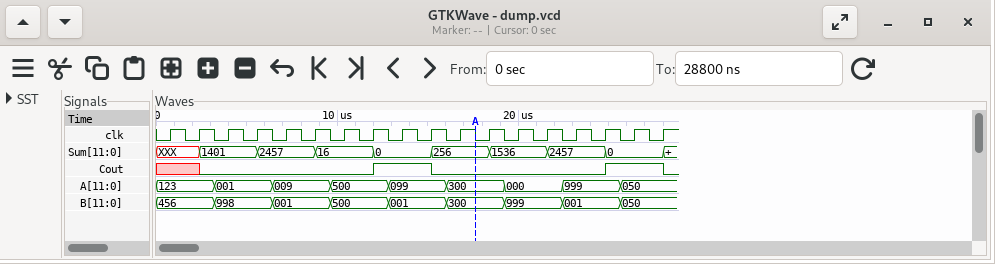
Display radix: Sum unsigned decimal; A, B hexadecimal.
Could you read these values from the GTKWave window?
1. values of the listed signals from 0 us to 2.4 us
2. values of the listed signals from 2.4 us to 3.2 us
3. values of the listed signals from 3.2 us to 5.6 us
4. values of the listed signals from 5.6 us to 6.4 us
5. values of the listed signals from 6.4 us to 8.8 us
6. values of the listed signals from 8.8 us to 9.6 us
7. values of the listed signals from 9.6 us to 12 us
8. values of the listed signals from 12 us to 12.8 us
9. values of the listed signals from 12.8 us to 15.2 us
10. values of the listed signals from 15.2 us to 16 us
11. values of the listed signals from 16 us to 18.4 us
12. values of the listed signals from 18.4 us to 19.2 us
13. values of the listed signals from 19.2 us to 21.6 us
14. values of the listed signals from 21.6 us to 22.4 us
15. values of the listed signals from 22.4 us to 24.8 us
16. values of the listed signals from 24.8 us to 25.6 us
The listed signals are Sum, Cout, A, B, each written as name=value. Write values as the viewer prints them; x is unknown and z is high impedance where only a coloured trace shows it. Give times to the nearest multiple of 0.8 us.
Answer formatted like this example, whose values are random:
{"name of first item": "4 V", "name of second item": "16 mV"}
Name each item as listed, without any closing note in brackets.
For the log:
{"values of the listed signals from 0 us to 2.4 us": "Sum=XXX, Cout=x, A=123, B=456", "values of the listed signals from 2.4 us to 3.2 us": "Sum=1401, Cout=0, A=123, B=456", "values of the listed signals from 3.2 us to 5.6 us": "Sum=1401, Cout=0, A=001, B=998", "values of the listed signals from 5.6 us to 6.4 us": "Sum=2457, Cout=0, A=001, B=998", "values of the listed signals from 6.4 us to 8.8 us": "Sum=2457, Cout=0, A=009, B=001", "values of the listed signals from 8.8 us to 9.6 us": "Sum=16, Cout=0, A=009, B=001", "values of the listed signals from 9.6 us to 12 us": "Sum=16, Cout=0, A=500, B=500", "values of the listed signals from 12 us to 12.8 us": "Sum=0, Cout=1, A=500, B=500", "values of the listed signals from 12.8 us to 15.2 us": "Sum=0, Cout=1, A=099, B=001", "values of the listed signals from 15.2 us to 16 us": "Sum=256, Cout=0, A=099, B=001", "values of the listed signals from 16 us to 18.4 us": "Sum=256, Cout=0, A=300, B=300", "values of the listed signals from 18.4 us to 19.2 us": "Sum=1536, Cout=0, A=300, B=300", "values of the listed signals from 19.2 us to 21.6 us": "Sum=1536, Cout=0, A=000, B=999", "values of the listed signals from 21.6 us to 22.4 us": "Sum=2457, Cout=0, A=000, B=999", "values of the listed signals from 22.4 us to 24.8 us": "Sum=2457, Cout=0, A=999, B=001", "values of the listed signals from 24.8 us to 25.6 us": "Sum=0, Cout=1, A=999, B=001"}
